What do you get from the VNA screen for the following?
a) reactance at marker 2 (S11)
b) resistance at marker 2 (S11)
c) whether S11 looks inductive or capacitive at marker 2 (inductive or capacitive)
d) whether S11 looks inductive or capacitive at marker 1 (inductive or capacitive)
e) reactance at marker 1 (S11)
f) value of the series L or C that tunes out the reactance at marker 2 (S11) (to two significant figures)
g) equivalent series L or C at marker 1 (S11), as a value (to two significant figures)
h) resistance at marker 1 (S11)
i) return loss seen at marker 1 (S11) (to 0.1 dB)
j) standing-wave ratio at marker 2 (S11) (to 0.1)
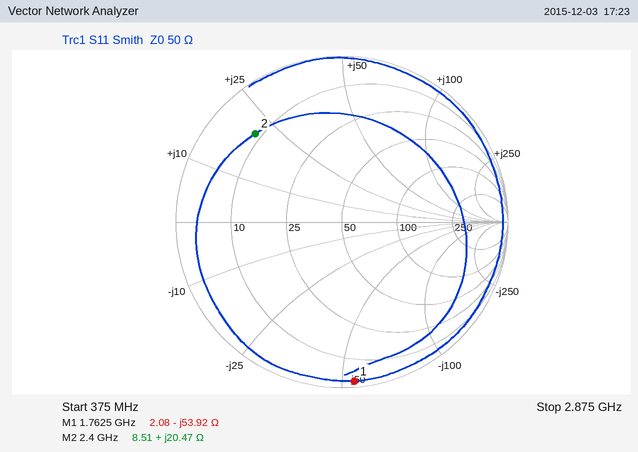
+20.47 Ω
8.51 Ω
inductive
capacitive
-53.92 Ω
3.2 pF
1.7 pF
2.08 Ω
0.3 dB
6.9
